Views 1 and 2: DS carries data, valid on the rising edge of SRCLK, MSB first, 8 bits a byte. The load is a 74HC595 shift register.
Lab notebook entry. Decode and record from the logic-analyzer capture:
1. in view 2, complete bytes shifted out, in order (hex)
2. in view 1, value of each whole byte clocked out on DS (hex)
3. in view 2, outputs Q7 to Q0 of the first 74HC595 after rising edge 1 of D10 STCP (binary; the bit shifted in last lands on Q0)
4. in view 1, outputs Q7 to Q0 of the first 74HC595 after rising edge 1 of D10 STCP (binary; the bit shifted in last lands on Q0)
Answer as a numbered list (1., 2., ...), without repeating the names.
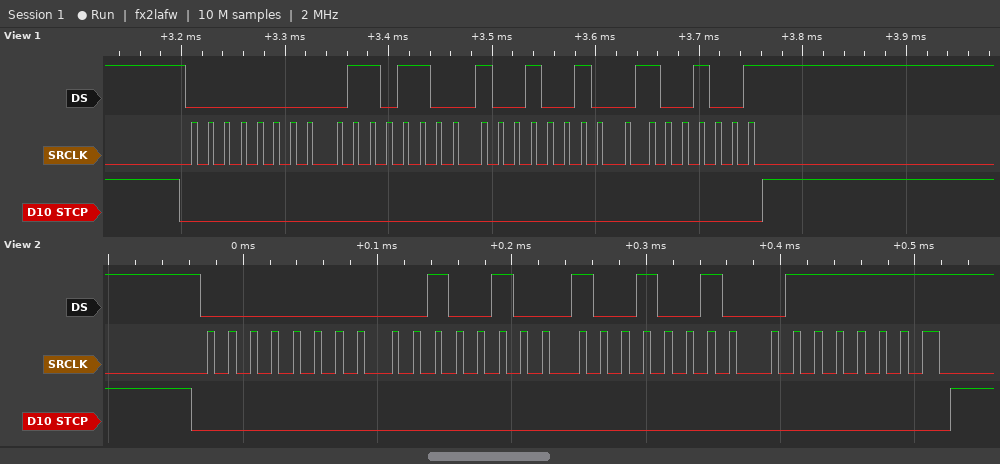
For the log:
1. 00 24 92 7F
2. 00 6C 92 49
3. 01111111
4. 01001001
